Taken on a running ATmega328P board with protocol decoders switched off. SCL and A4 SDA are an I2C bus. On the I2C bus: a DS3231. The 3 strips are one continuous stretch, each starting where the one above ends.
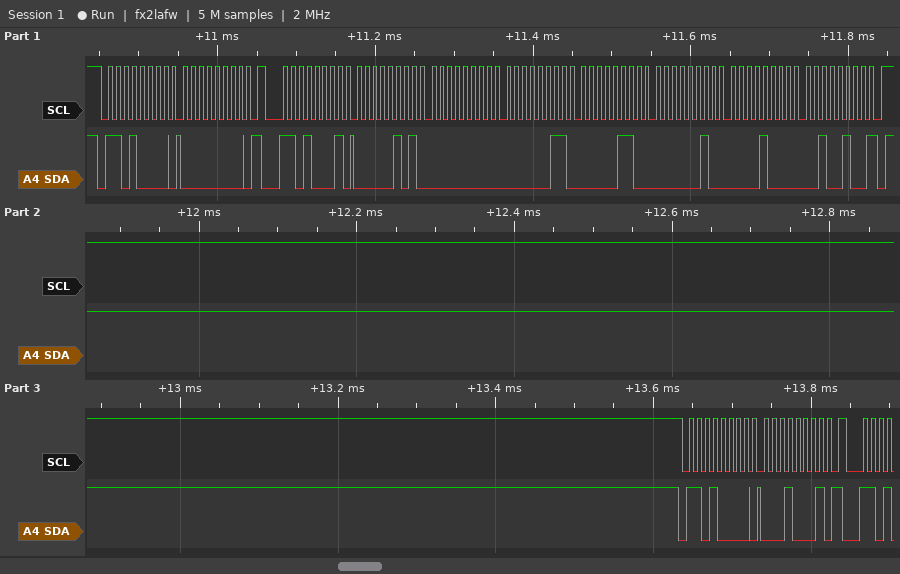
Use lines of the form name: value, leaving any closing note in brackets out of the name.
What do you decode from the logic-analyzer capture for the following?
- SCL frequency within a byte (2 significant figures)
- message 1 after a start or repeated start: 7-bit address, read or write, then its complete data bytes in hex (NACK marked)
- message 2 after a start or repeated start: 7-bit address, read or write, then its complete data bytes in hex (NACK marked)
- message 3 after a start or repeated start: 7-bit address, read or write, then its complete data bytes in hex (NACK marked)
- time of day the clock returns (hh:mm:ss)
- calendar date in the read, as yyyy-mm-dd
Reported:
SCL frequency within a byte: 100 kHz
message 1 after a start or repeated start: 7-bit address, read or write, then its complete data bytes in hex: 0x68 write: 00
message 2 after a start or repeated start: 7-bit address, read or write, then its complete data bytes in hex: 0x68 read: 05 00 03 06 02 08 24 NACK
message 3 after a start or repeated start: 7-bit address, read or write, then its complete data bytes in hex: 0x68 write: 11
time of day the clock returns: 03:00:05
calendar date in the read, as yyyy-mm-dd: 2024-08-02
